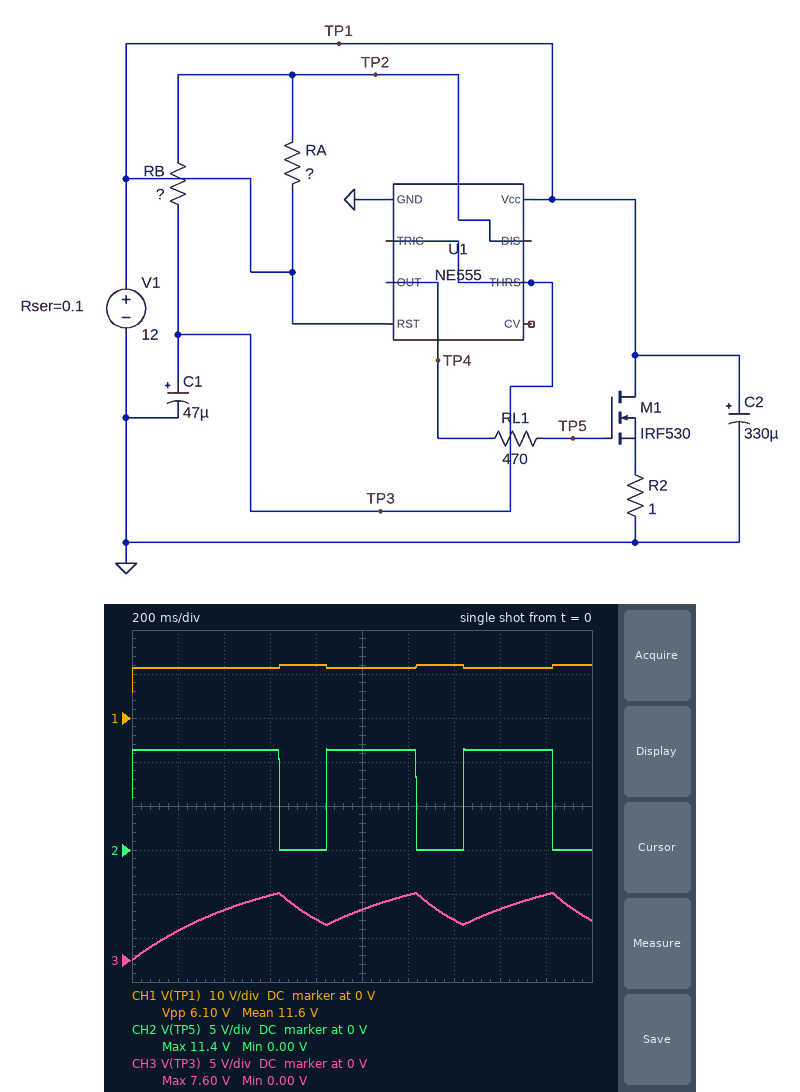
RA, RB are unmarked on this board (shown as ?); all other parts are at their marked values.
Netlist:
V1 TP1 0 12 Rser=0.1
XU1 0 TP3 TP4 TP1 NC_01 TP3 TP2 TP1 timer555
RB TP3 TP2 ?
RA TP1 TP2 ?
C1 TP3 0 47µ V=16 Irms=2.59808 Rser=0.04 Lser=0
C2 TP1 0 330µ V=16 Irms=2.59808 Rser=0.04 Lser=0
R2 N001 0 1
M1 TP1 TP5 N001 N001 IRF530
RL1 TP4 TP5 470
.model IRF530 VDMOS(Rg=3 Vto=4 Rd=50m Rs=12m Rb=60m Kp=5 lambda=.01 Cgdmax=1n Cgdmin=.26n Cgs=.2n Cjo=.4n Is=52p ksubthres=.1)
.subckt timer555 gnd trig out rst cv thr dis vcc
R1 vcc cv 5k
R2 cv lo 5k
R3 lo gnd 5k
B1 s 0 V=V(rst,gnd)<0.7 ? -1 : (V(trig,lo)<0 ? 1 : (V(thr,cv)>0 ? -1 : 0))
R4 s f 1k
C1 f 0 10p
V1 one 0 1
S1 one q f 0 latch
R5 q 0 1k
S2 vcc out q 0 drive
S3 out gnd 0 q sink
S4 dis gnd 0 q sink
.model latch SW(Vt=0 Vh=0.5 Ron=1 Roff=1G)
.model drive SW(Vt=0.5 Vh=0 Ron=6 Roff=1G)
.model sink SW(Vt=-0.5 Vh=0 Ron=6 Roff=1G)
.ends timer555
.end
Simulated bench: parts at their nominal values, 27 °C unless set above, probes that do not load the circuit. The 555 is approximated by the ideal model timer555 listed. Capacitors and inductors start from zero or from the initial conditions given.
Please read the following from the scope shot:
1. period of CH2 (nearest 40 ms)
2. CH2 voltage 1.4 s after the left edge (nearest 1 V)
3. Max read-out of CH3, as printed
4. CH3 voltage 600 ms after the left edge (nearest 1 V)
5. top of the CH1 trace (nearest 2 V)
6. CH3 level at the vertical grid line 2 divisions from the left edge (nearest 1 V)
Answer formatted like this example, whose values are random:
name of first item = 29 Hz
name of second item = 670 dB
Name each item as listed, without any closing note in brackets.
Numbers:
period of CH2 = 600 ms
CH2 voltage 1.4 s after the left edge = 0 V
Max read-out of CH3, as printed = 7.60 V
CH3 voltage 600 ms after the left edge = 7 V
top of the CH1 trace = 12 V
CH3 level at the vertical grid line 2 divisions from the left edge = 6 V
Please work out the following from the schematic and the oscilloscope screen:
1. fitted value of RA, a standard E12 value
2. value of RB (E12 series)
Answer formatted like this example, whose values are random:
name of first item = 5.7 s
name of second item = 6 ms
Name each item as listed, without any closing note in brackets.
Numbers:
fitted value of RA, a standard E12 value = 5.6 kΩ
value of RB = 6.8 kΩ
